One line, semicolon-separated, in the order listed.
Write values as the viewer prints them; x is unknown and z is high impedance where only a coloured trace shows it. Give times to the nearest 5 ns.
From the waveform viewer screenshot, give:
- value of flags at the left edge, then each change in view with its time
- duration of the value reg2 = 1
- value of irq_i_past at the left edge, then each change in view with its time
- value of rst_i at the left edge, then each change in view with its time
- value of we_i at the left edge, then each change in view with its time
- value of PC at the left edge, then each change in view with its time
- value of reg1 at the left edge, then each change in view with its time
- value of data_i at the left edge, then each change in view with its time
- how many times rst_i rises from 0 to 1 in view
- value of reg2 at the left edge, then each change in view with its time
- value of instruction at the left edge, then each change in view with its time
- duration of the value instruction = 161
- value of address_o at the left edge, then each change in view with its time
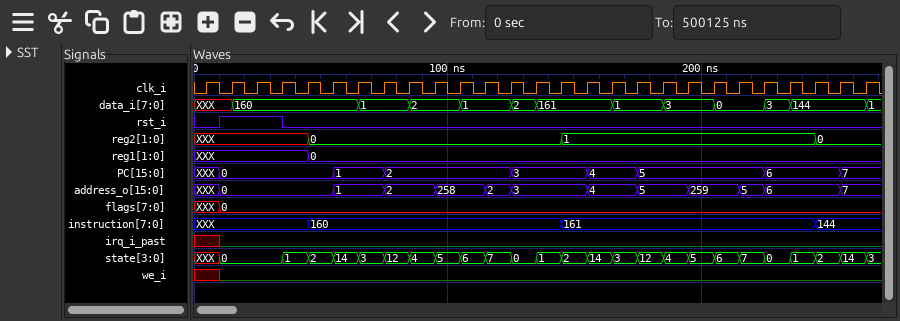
XXX, 0 at 10 ns; 100 ns; x, 0 at 10 ns; 0, 1 at 10 ns, 0 at 35 ns; x, 0 at 10 ns; XXX, 0 at 10 ns, 1 at 55 ns, 2 at 75 ns, 3 at 125 ns, 4 at 155 ns, 5 at 175 ns, 6 at 225 ns, 7 at 255 ns; XXX, 0 at 45 ns; XXX, 160 at 15 ns, 1 at 65 ns, 2 at 85 ns, 1 at 105 ns, 2 at 125 ns, 161 at 135 ns, 1 at 165 ns, 3 at 185 ns, 0 at 205 ns, 3 at 225 ns, 144 at 235 ns, 1 at 265 ns; 1; XXX, 0 at 45 ns, 1 at 145 ns, 0 at 245 ns; XXX, 160 at 45 ns, 161 at 145 ns, 144 at 245 ns; 100 ns; XXX, 0 at 10 ns, 1 at 55 ns, 2 at 75 ns, 258 at 95 ns, 2 at 115 ns, 3 at 125 ns, 4 at 155 ns, 5 at 175 ns, 259 at 195 ns, 5 at 215 ns, 6 at 225 ns, 7 at 255 ns
